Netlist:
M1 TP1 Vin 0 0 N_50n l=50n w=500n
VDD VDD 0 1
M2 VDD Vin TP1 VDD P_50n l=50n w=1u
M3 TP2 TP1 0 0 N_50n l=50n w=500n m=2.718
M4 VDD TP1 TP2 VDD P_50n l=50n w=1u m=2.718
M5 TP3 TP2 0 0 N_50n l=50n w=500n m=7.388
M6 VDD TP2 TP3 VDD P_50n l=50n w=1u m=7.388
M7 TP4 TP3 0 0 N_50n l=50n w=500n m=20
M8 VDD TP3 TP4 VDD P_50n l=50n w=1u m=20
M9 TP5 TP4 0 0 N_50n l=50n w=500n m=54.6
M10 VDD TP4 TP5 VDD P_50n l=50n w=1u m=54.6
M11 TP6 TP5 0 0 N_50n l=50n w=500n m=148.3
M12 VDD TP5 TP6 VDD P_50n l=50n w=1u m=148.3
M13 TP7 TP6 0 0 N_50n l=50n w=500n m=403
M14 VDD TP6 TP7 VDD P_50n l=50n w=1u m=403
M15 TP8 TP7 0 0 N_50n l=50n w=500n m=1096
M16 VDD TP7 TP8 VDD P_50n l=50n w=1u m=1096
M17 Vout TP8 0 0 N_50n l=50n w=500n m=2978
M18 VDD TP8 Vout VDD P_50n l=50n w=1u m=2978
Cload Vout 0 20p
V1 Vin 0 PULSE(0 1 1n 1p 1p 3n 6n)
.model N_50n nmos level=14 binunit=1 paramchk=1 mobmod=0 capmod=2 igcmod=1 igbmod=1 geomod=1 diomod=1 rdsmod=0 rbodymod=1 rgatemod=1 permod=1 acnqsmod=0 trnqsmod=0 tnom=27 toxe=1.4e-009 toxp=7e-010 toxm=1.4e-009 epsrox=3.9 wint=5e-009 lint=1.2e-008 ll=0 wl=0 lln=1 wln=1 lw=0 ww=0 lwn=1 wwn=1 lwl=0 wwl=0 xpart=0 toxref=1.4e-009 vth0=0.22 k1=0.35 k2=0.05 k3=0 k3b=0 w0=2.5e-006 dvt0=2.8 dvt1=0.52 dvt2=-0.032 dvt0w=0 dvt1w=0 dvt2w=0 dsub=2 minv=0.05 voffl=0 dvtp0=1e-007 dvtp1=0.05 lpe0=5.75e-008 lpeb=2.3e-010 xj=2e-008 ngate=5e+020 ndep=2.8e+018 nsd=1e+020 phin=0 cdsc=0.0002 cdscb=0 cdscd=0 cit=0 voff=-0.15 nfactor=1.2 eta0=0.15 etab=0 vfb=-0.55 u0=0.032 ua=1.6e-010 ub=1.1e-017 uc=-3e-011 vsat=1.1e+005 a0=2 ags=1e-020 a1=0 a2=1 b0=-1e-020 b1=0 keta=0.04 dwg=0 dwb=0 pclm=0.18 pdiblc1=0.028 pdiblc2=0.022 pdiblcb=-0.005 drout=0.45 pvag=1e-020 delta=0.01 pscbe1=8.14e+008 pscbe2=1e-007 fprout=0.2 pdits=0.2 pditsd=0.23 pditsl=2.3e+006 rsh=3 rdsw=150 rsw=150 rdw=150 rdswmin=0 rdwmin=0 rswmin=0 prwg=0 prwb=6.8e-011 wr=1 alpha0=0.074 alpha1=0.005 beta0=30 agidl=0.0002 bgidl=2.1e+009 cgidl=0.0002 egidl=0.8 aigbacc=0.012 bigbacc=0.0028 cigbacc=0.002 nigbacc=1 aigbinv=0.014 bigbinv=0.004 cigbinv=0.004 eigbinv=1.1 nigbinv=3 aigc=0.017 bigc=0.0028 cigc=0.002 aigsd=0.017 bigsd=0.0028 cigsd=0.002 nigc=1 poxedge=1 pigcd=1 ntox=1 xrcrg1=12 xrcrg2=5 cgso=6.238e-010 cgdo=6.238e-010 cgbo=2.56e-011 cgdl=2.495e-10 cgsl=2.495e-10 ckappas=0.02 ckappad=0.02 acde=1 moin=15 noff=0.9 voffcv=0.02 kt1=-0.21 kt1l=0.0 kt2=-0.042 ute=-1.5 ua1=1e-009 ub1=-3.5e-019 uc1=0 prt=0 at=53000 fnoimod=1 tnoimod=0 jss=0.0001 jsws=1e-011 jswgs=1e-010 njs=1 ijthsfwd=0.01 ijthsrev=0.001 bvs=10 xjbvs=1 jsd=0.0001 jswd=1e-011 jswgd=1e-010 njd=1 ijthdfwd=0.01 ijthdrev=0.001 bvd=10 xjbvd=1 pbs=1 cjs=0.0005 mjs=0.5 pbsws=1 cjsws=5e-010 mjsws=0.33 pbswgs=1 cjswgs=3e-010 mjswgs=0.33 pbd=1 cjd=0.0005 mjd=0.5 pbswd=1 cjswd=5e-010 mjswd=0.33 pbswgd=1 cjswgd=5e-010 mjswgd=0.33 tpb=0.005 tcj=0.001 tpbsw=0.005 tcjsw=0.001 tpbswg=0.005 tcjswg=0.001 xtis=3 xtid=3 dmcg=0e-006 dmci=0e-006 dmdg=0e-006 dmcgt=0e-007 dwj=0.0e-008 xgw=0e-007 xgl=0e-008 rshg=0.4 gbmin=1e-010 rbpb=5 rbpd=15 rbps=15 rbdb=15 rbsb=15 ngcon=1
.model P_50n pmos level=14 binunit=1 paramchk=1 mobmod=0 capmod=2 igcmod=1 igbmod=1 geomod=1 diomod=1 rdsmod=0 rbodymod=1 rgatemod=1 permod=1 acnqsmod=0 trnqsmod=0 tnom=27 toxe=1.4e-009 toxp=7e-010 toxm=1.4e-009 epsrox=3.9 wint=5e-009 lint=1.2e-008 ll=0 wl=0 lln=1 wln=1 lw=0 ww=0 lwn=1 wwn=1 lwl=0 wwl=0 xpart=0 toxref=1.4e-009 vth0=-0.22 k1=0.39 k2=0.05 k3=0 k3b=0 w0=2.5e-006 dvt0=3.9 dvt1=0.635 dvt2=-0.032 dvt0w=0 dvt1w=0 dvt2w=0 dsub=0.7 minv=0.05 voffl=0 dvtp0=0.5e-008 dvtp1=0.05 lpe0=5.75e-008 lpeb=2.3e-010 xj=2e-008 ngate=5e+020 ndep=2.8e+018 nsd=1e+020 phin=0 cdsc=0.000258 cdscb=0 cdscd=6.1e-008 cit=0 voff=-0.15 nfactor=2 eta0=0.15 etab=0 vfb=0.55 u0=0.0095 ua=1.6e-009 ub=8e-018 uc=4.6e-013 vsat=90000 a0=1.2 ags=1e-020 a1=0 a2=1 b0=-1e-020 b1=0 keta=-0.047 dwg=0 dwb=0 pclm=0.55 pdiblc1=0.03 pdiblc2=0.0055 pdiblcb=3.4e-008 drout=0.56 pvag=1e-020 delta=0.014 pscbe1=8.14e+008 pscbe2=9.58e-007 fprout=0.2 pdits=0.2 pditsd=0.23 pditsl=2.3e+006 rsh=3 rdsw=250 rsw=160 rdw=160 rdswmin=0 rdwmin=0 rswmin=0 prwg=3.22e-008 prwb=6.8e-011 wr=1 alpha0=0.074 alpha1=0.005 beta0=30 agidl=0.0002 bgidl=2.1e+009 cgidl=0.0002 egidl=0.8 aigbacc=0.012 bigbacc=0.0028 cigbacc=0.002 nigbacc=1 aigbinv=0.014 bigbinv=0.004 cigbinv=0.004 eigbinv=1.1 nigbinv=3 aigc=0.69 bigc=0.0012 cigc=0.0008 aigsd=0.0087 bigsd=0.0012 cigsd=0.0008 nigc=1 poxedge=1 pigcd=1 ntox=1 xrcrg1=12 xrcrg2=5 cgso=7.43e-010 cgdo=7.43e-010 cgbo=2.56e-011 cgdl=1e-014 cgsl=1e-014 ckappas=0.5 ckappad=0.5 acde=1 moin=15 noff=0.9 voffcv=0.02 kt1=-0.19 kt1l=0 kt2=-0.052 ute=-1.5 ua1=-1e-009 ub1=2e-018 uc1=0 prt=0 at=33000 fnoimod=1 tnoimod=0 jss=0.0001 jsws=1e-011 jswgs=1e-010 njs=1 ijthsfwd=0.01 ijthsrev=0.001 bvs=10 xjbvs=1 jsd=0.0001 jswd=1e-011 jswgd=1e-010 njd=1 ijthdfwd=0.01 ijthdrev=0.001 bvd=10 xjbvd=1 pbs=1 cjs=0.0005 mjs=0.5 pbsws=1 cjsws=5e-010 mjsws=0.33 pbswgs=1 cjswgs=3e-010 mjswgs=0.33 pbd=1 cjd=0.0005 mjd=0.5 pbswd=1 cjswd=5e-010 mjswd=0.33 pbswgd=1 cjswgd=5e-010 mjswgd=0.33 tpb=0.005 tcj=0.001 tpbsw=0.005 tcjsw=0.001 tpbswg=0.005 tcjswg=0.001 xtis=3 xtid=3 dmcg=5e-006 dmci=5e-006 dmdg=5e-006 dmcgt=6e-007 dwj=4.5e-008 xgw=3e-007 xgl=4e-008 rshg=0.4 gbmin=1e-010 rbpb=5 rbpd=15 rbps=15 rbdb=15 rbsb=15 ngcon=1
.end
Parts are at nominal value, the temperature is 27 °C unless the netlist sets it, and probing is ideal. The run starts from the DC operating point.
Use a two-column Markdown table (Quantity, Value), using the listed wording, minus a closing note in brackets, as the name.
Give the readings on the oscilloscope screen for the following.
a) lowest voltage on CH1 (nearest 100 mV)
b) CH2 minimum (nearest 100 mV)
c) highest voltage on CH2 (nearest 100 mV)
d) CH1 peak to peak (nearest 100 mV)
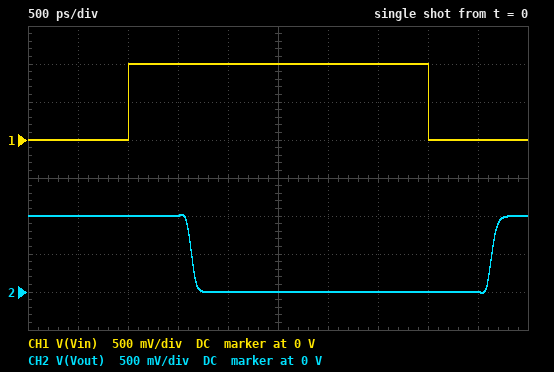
| Quantity | Value |
|---|---|
| lowest voltage on CH1 | 0 V |
| CH2 minimum | 0 V |
| highest voltage on CH2 | 1.0 V |
| CH1 peak to peak | 1.0 V |
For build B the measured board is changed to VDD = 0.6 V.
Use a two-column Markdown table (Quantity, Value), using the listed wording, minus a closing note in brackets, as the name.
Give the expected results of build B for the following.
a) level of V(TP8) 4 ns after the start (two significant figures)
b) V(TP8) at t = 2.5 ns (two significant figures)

| Quantity | Value |
|---|---|
| level of V(TP8) 4 ns after the start | 600 mV |
| V(TP8) at t = 2.5 ns | 580 mV |
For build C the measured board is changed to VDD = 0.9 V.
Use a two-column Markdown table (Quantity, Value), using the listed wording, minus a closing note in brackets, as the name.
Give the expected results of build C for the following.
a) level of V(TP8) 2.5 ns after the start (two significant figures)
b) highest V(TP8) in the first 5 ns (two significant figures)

| Quantity | Value |
|---|---|
| level of V(TP8) 2.5 ns after the start | 900 mV |
| highest V(TP8) in the first 5 ns | 910 mV |
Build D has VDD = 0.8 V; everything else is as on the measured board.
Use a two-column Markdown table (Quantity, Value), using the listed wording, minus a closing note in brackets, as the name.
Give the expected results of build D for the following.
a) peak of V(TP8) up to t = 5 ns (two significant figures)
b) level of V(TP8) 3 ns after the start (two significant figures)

| Quantity | Value |
|---|---|
| peak of V(TP8) up to t = 5 ns | 810 mV |
| level of V(TP8) 3 ns after the start | 800 mV |
